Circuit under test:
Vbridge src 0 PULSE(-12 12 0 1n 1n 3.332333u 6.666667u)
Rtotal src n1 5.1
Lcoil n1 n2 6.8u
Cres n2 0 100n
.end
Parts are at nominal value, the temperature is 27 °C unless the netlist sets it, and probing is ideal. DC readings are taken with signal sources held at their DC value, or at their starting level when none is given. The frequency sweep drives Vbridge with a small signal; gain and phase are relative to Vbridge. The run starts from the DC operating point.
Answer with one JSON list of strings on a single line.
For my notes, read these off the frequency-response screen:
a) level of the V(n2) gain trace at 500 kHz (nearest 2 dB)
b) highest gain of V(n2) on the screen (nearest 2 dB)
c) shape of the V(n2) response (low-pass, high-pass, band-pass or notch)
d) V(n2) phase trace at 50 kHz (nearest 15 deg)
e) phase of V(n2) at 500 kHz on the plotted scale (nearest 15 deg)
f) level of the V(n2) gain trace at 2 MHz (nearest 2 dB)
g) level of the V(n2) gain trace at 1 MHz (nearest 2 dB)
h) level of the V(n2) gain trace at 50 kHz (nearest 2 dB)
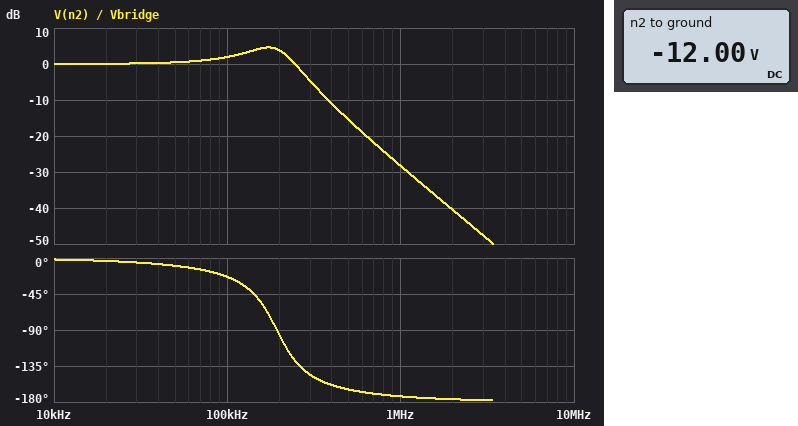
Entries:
["-16 dB", "4 dB", "low-pass", "-15 deg", "-165 deg", "-40 dB", "-28 dB", "0 dB"]
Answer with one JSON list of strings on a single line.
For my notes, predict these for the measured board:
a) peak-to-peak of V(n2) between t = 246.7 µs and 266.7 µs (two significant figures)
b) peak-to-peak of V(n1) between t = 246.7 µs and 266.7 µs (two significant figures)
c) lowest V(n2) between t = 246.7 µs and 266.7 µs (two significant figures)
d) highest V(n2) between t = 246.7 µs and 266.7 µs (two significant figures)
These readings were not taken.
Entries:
["47 V", "33 V", "-24 V", "24 V"]
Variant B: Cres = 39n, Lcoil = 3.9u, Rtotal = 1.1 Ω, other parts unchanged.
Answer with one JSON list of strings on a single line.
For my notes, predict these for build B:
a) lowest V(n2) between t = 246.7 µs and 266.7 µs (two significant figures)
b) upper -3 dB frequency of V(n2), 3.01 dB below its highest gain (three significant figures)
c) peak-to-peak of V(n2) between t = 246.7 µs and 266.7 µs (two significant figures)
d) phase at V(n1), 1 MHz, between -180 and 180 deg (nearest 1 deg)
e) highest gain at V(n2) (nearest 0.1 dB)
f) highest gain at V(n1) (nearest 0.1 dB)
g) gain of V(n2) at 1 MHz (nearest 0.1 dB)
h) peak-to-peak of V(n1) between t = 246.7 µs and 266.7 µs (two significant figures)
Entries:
["-37 V", "429 kHz", "74 V", "3 deg", "19.2 dB", "0 dB", "-14.0 dB", "29 V"]
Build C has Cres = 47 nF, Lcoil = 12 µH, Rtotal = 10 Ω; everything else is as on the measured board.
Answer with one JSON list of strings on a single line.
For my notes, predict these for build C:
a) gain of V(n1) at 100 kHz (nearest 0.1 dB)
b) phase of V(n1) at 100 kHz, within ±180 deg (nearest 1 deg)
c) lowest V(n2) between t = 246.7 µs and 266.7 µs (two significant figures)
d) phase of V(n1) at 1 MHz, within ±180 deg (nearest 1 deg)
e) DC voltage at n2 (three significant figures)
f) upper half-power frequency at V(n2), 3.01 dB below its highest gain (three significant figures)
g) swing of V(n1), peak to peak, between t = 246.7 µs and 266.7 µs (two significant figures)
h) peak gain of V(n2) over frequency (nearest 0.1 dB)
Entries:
["-0.6 dB", "-21 deg", "-22 V", "8 deg", "-12.0 V", "251 kHz", "32 V", "4.5 dB"]
